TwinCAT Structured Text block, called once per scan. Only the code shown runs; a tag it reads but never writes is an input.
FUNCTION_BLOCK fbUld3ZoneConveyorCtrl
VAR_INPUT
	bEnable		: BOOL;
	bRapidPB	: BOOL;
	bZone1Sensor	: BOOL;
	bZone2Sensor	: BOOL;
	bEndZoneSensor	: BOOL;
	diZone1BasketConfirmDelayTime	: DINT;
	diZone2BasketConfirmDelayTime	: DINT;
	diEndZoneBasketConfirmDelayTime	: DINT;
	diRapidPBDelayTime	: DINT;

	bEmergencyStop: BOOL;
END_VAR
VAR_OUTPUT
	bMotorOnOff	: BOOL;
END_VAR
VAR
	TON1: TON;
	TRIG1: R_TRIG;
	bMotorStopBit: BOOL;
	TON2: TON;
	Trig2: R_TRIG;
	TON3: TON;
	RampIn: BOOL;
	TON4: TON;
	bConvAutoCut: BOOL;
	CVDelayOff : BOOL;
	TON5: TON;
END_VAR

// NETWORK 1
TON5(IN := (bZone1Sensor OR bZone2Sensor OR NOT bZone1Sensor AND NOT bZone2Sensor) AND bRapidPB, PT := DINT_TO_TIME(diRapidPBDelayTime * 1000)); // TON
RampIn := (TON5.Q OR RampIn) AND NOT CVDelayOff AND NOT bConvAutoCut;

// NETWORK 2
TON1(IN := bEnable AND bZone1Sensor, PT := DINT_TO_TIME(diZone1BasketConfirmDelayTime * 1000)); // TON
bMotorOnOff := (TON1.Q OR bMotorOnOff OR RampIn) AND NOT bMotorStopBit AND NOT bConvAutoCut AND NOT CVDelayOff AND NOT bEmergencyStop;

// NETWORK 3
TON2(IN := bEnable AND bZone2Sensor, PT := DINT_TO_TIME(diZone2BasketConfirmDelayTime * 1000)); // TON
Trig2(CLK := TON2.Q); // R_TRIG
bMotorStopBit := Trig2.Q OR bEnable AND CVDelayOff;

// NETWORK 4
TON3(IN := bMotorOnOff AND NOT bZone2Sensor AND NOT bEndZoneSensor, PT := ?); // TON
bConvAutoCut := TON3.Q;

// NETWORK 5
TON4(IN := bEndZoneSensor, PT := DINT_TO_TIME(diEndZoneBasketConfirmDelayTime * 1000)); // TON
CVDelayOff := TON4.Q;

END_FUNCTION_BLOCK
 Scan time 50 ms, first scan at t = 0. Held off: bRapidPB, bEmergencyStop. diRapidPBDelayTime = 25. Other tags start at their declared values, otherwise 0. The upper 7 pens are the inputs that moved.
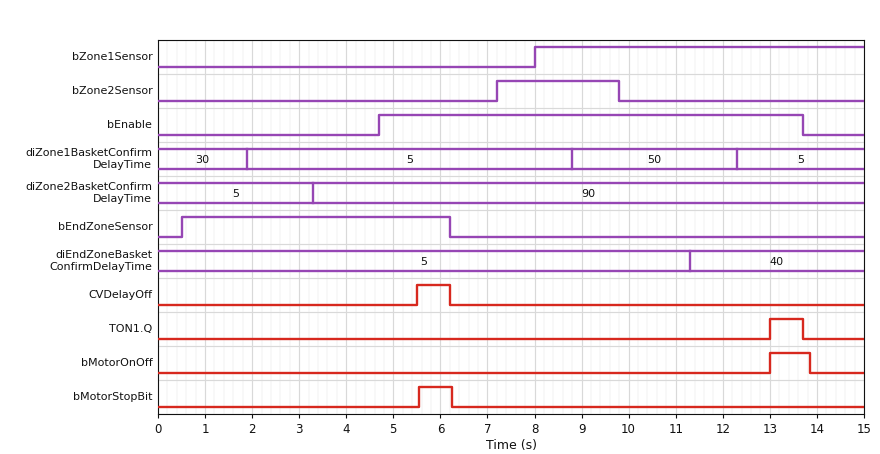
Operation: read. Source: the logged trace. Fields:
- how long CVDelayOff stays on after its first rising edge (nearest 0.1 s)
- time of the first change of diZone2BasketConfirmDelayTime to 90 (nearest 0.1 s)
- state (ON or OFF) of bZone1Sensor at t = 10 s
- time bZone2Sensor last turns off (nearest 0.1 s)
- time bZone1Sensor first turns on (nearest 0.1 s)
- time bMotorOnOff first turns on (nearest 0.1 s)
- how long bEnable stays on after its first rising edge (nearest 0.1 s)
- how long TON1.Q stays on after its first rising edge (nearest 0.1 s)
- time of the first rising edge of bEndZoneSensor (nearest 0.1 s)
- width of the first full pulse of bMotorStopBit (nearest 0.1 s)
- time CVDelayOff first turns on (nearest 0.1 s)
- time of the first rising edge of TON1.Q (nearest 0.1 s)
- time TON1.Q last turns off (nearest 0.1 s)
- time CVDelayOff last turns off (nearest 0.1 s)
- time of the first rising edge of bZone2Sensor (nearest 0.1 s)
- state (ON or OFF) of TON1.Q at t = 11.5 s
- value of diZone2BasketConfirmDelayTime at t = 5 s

0.7 s
3.3 s
ON
9.8 s
8.0 s
13.0 s
9.0 s
0.7 s
0.5 s
0.7 s
5.5 s
13.0 s
13.7 s
6.2 s
7.2 s
OFF
90
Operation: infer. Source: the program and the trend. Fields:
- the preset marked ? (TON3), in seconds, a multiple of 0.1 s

0.8 s
